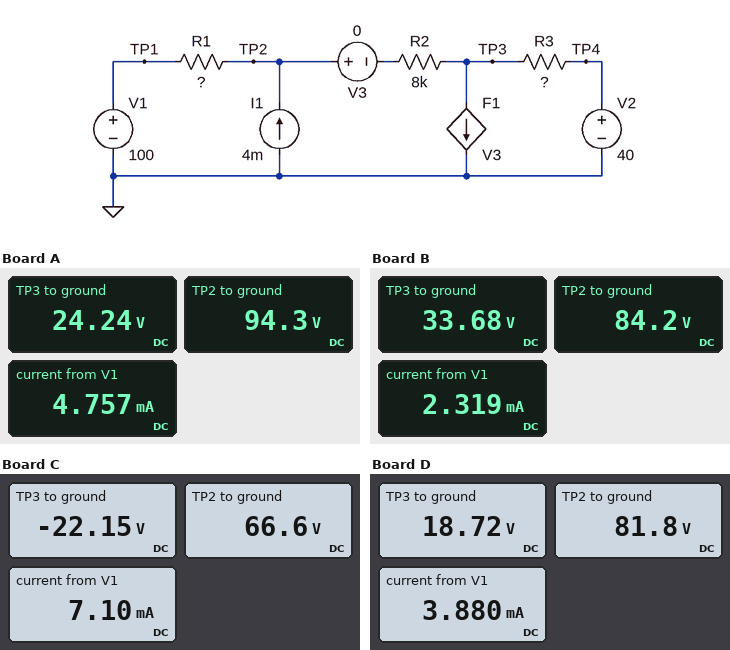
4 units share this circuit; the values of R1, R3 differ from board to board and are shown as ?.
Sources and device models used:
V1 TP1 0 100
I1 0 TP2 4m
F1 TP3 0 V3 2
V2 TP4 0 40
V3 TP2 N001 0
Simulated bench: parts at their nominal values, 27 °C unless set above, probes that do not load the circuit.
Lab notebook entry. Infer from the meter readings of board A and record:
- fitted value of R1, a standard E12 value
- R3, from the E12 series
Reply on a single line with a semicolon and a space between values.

1.2 kΩ; 1.8 kΩ
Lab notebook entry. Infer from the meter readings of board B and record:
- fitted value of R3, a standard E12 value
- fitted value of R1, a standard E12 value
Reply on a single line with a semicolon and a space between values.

1 kΩ; 6.8 kΩ
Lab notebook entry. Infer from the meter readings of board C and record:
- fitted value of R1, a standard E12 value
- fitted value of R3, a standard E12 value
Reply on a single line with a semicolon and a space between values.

4.7 kΩ; 5.6 kΩ
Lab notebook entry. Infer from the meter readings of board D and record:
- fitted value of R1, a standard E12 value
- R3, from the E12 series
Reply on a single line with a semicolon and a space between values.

4.7 kΩ; 2.7 kΩ
